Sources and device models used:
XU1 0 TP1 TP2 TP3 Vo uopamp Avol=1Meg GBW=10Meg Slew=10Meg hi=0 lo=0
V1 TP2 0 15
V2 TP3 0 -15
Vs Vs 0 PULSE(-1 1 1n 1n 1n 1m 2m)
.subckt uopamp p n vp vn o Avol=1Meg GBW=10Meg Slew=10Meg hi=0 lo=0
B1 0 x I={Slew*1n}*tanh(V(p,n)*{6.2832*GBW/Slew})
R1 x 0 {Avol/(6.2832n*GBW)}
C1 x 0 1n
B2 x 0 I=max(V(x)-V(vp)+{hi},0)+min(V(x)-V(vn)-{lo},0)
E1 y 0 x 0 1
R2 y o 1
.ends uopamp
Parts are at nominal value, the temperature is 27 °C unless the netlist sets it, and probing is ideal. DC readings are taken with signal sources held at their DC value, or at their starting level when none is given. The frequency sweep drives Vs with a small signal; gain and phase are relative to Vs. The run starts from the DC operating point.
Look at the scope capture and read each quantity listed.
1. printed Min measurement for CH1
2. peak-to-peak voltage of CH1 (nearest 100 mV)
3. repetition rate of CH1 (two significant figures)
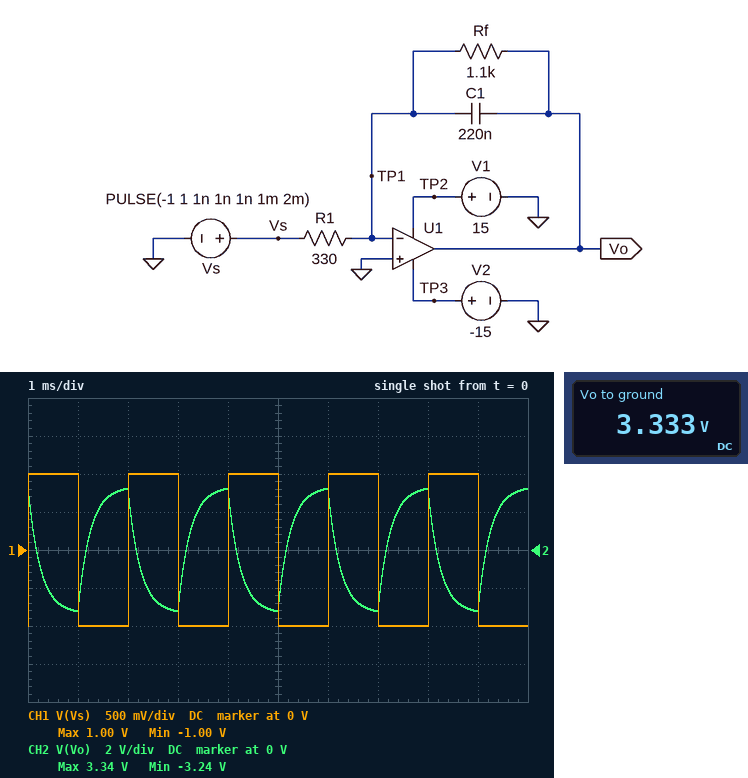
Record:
-1.00 V
2.0 V
500 Hz
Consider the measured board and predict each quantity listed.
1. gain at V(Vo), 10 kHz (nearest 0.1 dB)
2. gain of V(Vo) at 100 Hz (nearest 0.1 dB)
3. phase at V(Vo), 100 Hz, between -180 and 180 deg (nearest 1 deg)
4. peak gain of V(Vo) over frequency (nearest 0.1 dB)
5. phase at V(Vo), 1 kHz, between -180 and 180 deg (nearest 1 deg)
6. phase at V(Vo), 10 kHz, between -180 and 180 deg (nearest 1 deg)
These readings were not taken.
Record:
-13.2 dB
10.4 dB
171 deg
10.5 dB
123 deg
94 deg
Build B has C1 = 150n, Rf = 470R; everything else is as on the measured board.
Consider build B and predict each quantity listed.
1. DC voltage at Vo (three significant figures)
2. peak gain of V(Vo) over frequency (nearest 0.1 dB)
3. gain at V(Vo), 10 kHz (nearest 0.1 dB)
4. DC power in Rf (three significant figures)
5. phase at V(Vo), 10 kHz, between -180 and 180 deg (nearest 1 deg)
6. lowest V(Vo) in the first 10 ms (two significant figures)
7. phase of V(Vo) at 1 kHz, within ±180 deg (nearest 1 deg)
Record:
1.42 V
3.1 dB
-10.1 dB
4.32 mW
103 deg
-1.4 V
156 deg
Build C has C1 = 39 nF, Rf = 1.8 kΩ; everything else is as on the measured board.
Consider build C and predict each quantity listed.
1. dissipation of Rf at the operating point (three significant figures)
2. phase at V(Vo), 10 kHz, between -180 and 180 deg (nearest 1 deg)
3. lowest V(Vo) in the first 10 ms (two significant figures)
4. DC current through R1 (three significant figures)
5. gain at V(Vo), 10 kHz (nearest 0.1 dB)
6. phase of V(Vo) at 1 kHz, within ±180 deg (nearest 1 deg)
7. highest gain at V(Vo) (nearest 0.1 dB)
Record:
16.5 mW
103 deg
-5.5 V
3.03 mA
1.6 dB
156 deg
14.7 dB
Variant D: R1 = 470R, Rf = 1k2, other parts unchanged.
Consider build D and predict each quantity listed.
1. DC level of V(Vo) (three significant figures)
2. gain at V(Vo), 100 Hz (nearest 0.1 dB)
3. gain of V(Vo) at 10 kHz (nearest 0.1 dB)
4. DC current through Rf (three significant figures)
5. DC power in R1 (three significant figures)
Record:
2.55 V
8.0 dB
-16.3 dB
2.13 mA
2.13 mW
